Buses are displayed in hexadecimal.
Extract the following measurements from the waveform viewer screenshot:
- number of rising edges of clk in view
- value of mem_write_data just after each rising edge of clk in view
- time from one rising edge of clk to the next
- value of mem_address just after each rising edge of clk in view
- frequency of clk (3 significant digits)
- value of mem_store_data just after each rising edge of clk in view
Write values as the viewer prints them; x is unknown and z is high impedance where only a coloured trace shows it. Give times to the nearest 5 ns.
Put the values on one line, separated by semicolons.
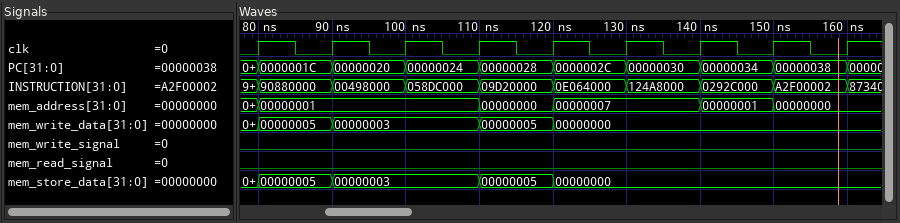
9; 00000005, 00000003, 00000003, 00000005, 00000000, 00000000, 00000000, 00000000, 00000000; 10 ns; 00000001, 00000001, 00000001, 00000000, 00000007, 00000007, 00000001, 00000000, 00000000; 100 MHz; 00000005, 00000003, 00000003, 00000005, 00000000, 00000000, 00000000, 00000000, 00000000
